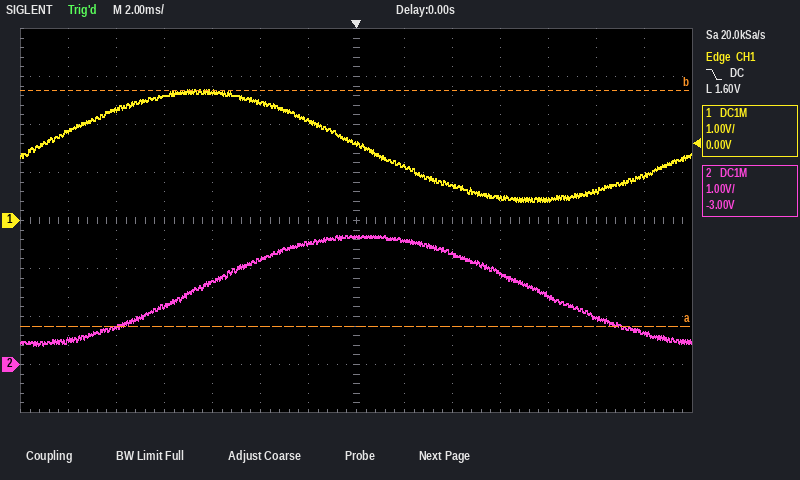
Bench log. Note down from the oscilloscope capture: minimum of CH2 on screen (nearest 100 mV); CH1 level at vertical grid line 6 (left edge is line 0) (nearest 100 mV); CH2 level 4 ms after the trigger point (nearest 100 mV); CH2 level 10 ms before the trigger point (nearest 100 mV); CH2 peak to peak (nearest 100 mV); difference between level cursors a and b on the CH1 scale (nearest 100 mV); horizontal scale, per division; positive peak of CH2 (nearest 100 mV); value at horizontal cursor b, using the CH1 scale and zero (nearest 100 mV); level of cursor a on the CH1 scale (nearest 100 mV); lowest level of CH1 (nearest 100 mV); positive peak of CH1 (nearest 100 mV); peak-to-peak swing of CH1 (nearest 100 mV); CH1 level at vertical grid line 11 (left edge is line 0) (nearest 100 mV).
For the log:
400 mV
2.1 V
2.3 V
800 mV
2.3 V
4.9 V
2 ms
2.7 V
2.7 V
-2.2 V
400 mV
2.7 V
2.3 V
400 mV
